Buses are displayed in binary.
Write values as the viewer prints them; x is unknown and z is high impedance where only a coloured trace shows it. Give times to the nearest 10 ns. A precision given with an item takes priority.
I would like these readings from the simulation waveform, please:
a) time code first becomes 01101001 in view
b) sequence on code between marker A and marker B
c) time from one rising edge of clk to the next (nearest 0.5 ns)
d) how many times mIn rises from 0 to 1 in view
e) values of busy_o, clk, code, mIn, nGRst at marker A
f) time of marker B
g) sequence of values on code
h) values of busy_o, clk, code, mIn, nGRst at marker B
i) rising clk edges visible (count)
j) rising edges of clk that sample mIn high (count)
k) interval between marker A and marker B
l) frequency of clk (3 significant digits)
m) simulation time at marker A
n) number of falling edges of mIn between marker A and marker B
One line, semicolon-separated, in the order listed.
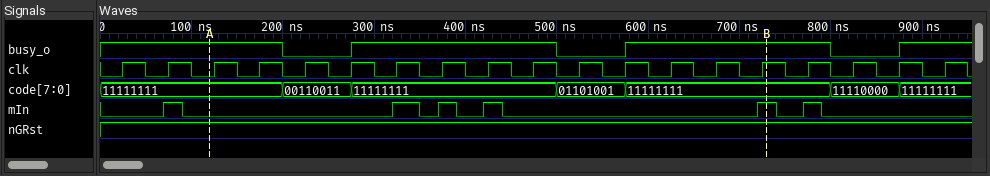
500 ns; 11111111, 00110011, 11111111, 01101001, 11111111; 50 ns; 6; busy_o=1, clk=0, code=11111111, mIn=0, nGRst=1; 730 ns; 11111111, 00110011, 11111111, 01101001, 11111111, 11110000, 11111111; busy_o=1, clk=1, code=11111111, mIn=1, nGRst=1; 19; 6; 610 ns; 20.0 MHz; 120 ns; 3
